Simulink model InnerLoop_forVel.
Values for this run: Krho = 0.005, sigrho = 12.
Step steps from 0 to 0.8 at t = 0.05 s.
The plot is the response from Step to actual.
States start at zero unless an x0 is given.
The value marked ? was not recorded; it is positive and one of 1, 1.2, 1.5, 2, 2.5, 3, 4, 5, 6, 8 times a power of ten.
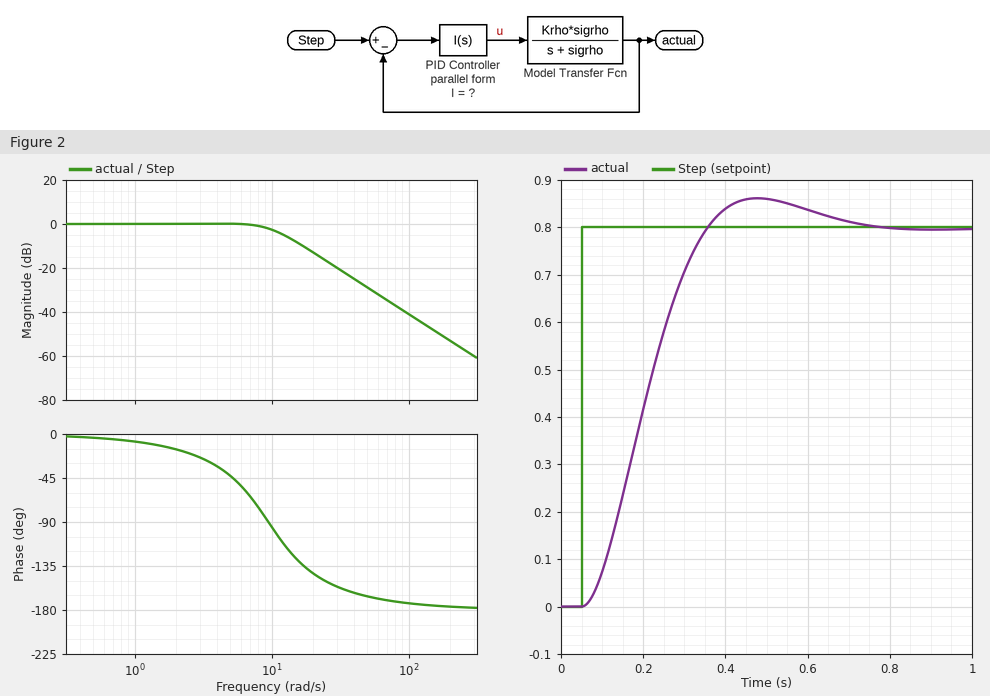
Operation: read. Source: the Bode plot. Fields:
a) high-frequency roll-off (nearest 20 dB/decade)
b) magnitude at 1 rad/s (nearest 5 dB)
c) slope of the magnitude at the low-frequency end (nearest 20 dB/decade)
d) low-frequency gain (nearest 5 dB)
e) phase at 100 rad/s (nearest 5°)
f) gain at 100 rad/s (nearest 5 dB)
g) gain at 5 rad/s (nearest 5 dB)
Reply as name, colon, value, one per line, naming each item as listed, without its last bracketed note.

high-frequency roll-off: -40 dB/decade
magnitude at 1 rad/s: 0 dB
slope of the magnitude at the low-frequency end: 0 dB/decade
low-frequency gain: 0 dB
phase at 100 rad/s: -175°
gain at 100 rad/s: -40 dB
gain at 5 rad/s: 0 dB
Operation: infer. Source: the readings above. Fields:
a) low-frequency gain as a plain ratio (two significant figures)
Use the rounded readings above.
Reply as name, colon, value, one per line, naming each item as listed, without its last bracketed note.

low-frequency gain as a plain ratio: 1.0
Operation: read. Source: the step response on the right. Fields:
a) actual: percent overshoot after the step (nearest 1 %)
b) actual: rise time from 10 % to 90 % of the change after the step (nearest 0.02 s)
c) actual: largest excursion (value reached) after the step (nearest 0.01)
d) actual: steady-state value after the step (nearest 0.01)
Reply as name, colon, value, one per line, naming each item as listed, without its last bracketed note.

actual: percent overshoot after the step: 8 %
actual: rise time from 10 % to 90 % of the change after the step: 0.20 s
actual: largest excursion (value reached) after the step: 0.86
actual: steady-state value after the step: 0.80
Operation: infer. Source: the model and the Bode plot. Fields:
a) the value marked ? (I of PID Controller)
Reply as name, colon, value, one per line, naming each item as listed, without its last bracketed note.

the value marked ?: 1500
